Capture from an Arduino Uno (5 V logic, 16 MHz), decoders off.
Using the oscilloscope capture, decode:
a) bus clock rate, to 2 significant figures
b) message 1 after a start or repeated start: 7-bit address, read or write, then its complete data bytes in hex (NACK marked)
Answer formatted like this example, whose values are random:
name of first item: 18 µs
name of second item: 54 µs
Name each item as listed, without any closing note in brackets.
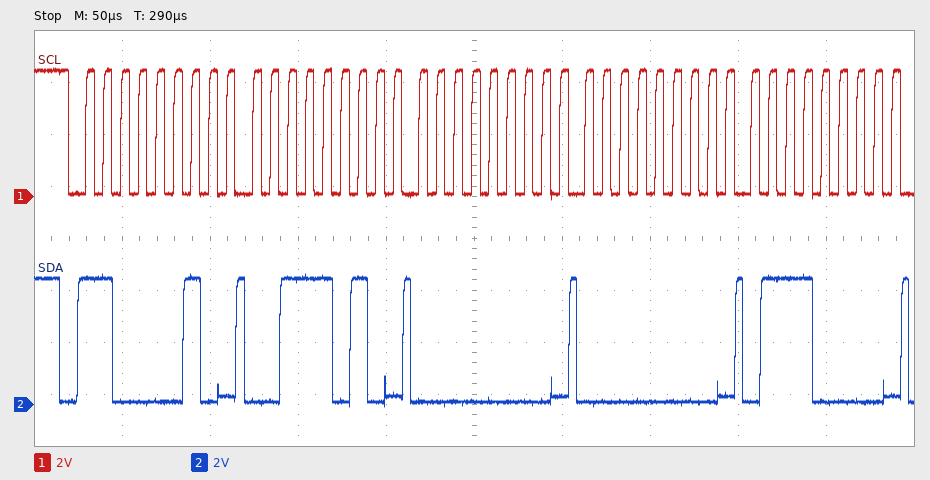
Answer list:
bus clock rate, to 2 significant figures: 100 kHz
message 1 after a start or repeated start: 7-bit address, read or write, then its complete data bytes in hex: 0x61 write: 3A 00 00 70
